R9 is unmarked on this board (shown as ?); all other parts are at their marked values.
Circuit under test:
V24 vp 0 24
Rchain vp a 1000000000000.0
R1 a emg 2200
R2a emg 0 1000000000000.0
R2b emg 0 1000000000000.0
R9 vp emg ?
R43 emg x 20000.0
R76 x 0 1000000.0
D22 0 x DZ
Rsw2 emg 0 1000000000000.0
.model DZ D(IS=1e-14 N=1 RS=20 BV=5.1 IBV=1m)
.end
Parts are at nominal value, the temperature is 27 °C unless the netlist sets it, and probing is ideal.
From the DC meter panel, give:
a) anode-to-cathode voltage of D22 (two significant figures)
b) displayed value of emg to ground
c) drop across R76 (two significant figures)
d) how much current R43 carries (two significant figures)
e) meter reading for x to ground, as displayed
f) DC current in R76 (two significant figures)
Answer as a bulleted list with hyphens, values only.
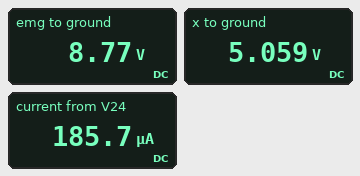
- -5.1 V
- 8.77 V
- 5.1 V
- 190 µA
- 5.059 V
- 5.1 µA
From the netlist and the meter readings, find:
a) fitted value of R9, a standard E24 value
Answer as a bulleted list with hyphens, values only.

- 82 kΩ
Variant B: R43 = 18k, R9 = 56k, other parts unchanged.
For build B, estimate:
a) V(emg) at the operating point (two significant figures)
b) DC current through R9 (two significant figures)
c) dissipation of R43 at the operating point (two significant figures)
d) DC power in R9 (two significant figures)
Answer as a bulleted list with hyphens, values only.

- 9.7 V
- 260 µA
- 1.2 mW
- 3.7 mW
